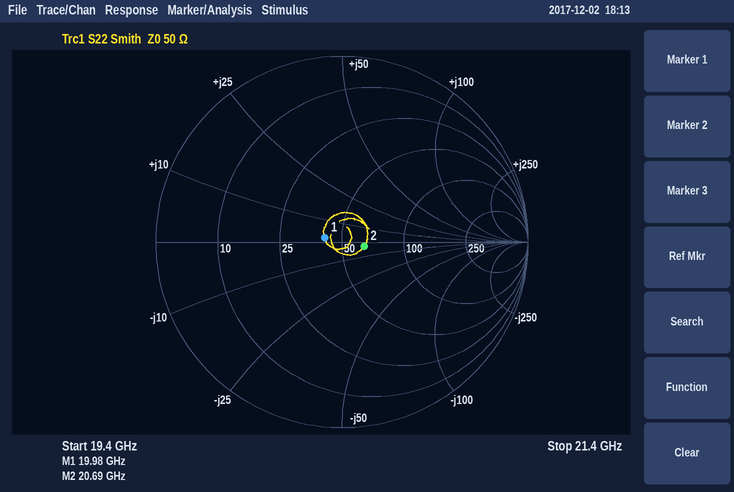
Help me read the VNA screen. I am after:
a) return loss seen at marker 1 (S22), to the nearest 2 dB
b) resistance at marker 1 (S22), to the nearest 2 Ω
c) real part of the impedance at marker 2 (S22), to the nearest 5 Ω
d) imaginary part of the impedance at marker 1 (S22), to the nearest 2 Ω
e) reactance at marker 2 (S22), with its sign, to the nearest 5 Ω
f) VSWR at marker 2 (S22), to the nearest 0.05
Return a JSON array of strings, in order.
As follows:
["20 dB", "42 Ω", "65 Ω", "+2 Ω", "-5 Ω", "1.30"]
